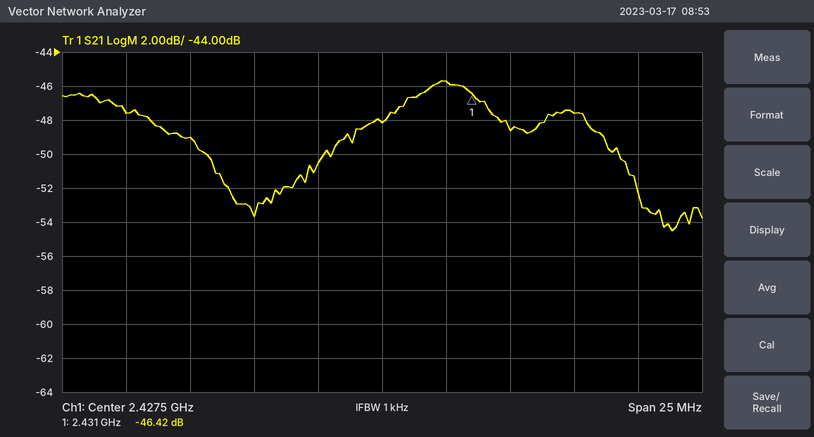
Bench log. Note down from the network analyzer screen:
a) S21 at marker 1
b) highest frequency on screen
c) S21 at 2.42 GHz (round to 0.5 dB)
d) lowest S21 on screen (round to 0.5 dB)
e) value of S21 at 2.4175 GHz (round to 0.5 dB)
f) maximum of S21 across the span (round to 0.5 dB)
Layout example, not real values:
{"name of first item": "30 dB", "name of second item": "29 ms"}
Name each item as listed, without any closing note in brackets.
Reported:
{"S21 at marker 1": "-46.42 dB", "highest frequency on screen": "2.44 GHz", "S21 at 2.42 GHz": "-49.0 dB", "lowest S21 on screen": "-54.5 dB", "value of S21 at 2.4175 GHz": "-47.5 dB", "maximum of S21 across the span": "-45.5 dB"}
